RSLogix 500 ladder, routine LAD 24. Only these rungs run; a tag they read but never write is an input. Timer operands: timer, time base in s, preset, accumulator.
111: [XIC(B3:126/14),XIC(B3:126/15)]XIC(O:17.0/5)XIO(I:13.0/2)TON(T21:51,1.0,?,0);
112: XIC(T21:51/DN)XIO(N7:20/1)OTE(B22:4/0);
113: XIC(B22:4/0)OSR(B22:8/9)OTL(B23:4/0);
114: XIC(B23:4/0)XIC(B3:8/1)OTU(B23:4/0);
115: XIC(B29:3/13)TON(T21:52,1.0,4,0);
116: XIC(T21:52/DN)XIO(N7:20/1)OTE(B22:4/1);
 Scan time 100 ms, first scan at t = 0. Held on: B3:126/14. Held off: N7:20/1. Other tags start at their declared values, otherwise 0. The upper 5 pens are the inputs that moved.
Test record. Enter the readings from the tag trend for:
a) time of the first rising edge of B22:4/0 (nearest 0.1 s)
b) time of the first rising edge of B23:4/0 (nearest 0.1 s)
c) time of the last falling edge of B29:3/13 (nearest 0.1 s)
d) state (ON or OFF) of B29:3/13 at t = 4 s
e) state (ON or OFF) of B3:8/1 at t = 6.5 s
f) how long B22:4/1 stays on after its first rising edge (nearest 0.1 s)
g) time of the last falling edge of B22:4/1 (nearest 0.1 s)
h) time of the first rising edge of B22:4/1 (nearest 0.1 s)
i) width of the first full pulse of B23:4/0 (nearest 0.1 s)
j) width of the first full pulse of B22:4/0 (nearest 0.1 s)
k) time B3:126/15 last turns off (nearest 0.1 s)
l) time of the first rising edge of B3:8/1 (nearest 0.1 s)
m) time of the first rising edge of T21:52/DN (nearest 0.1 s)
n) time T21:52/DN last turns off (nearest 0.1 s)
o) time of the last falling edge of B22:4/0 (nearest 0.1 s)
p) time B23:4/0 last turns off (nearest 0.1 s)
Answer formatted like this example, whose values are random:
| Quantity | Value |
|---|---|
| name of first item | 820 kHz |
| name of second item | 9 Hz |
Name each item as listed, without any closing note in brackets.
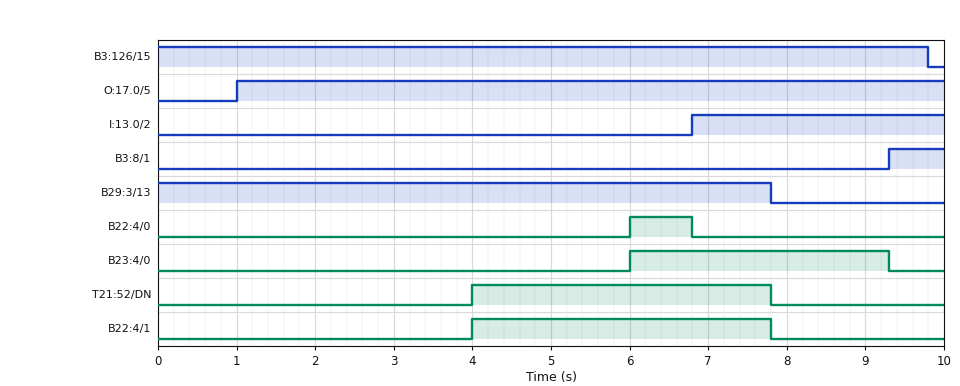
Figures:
| Quantity | Value |
|---|---|
| time of the first rising edge of B22:4/0 | 6.0 s |
| time of the first rising edge of B23:4/0 | 6.0 s |
| time of the last falling edge of B29:3/13 | 7.8 s |
| state (ON or OFF) of B29:3/13 at t = 4 s | ON |
| state (ON or OFF) of B3:8/1 at t = 6.5 s | OFF |
| how long B22:4/1 stays on after its first rising edge | 3.8 s |
| time of the last falling edge of B22:4/1 | 7.8 s |
| time of the first rising edge of B22:4/1 | 4.0 s |
| width of the first full pulse of B23:4/0 | 3.3 s |
| width of the first full pulse of B22:4/0 | 0.8 s |
| time B3:126/15 last turns off | 9.8 s |
| time of the first rising edge of B3:8/1 | 9.3 s |
| time of the first rising edge of T21:52/DN | 4.0 s |
| time T21:52/DN last turns off | 7.8 s |
| time of the last falling edge of B22:4/0 | 6.8 s |
| time B23:4/0 last turns off | 9.3 s |
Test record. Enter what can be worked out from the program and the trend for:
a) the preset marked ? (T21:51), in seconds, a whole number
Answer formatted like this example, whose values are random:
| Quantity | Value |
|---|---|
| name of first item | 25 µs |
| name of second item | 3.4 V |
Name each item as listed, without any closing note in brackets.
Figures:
| Quantity | Value |
|---|---|
| the preset marked ? (T21:51), in seconds, a whole number | 5 s |
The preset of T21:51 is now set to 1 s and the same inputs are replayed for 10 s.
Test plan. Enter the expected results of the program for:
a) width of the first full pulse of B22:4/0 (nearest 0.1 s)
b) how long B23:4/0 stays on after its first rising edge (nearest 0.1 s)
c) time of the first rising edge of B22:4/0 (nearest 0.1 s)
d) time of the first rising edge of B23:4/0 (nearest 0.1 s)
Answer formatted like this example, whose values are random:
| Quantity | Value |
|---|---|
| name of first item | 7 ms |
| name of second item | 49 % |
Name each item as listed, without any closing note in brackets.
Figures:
| Quantity | Value |
|---|---|
| width of the first full pulse of B22:4/0 | 4.8 s |
| how long B23:4/0 stays on after its first rising edge | 7.3 s |
| time of the first rising edge of B22:4/0 | 2.0 s |
| time of the first rising edge of B23:4/0 | 2.0 s |
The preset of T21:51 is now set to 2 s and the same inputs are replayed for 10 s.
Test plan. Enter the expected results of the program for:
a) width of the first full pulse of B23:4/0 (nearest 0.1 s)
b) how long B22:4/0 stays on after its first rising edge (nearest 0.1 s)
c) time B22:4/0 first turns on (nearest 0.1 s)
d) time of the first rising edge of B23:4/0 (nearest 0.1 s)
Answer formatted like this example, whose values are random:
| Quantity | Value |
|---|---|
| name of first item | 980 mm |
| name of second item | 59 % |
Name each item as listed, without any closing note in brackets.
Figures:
| Quantity | Value |
|---|---|
| width of the first full pulse of B23:4/0 | 6.3 s |
| how long B22:4/0 stays on after its first rising edge | 3.8 s |
| time B22:4/0 first turns on | 3.0 s |
| time of the first rising edge of B23:4/0 | 3.0 s |
